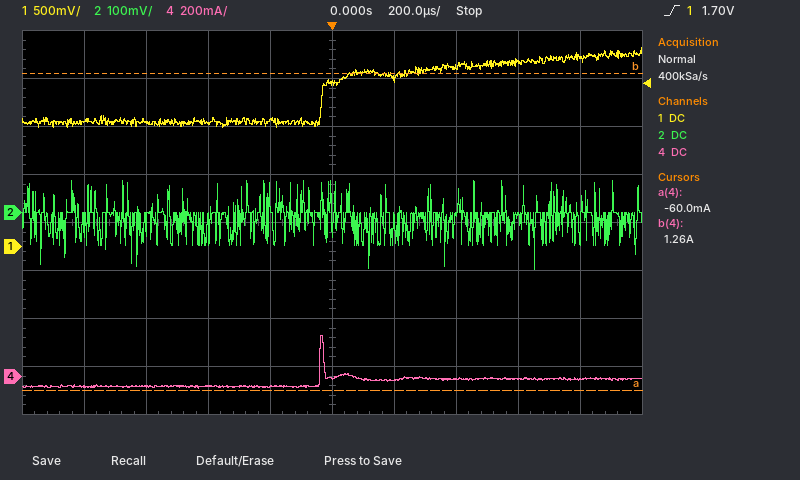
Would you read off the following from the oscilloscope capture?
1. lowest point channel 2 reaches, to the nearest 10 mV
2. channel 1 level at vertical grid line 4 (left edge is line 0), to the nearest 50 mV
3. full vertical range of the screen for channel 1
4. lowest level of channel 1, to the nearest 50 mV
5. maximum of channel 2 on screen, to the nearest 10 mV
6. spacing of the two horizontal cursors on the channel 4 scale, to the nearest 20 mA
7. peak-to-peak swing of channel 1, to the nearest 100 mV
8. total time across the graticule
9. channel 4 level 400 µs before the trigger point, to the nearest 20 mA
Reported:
-120 mV
1.30 V
4 V
1.25 V
70 mV
1.32 A
800 mV
2 ms
-40 mA
